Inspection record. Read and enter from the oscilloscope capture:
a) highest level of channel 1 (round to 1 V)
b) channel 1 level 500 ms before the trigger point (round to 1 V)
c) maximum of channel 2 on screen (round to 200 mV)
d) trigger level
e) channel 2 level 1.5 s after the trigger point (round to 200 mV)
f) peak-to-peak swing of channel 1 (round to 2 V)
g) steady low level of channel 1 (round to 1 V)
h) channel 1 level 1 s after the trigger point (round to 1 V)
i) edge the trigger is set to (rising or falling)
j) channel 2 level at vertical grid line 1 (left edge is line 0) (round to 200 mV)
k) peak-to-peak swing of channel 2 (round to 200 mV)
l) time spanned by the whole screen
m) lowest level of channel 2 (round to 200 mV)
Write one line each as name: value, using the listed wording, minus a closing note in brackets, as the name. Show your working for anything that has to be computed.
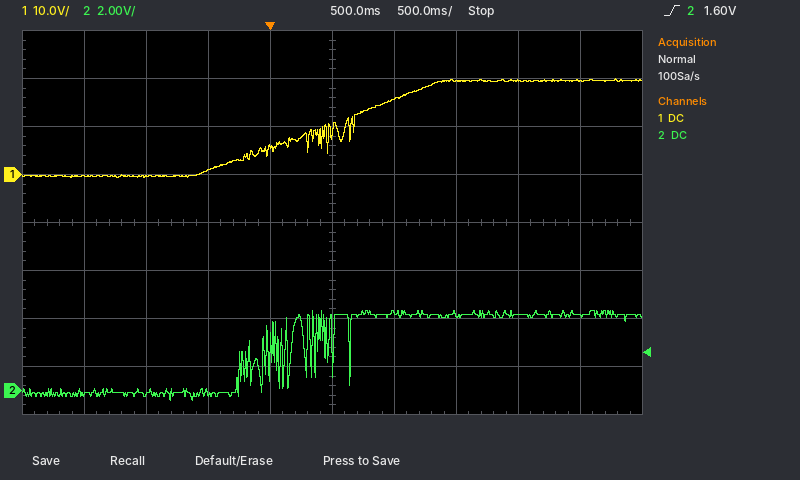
highest level of channel 1: 20 V
channel 1 level 500 ms before the trigger point: 1 V
maximum of channel 2 on screen: 3.4 V
trigger level: 1.60 V
channel 2 level 1.5 s after the trigger point: 3.2 V
peak-to-peak swing of channel 1: 20 V
steady low level of channel 1: 0 V
channel 1 level 1 s after the trigger point: 16 V
edge the trigger is set to: rising
channel 2 level at vertical grid line 1 (left edge is line 0): -200 mV
peak-to-peak swing of channel 2: 3.4 V − (-400 mV) = 3.8 V
time spanned by the whole screen: 5 s
lowest level of channel 2: -400 mV
